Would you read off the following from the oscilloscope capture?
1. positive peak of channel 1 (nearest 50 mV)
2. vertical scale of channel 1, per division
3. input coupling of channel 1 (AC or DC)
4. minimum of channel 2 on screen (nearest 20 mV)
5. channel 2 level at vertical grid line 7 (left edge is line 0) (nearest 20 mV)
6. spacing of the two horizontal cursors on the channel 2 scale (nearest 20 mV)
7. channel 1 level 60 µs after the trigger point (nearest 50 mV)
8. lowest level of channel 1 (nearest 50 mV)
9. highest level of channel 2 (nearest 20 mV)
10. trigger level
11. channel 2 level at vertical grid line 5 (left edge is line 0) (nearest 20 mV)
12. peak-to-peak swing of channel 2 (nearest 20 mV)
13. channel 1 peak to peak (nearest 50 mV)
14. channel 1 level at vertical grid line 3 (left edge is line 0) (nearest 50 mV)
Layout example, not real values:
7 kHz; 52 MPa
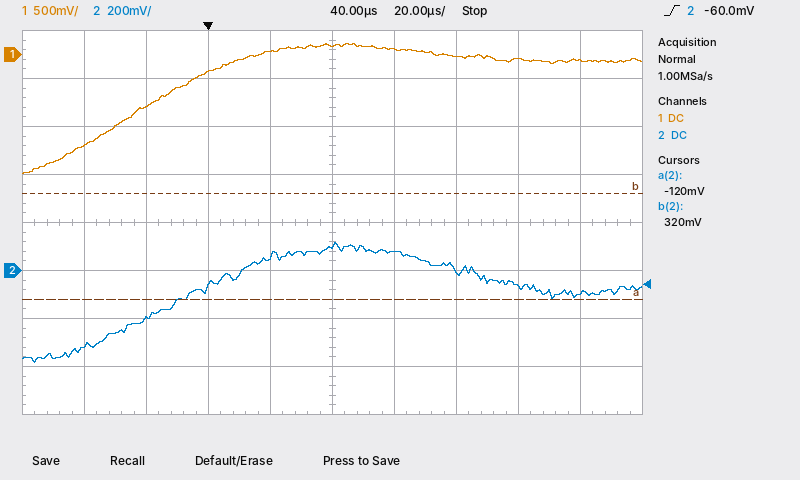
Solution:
100 mV; 500 mV; DC; -380 mV; 0 mV; 440 mV; 50 mV; -1.25 V; 120 mV; -60.0 mV; 100 mV; 500 mV; 1.35 V; -200 mV
